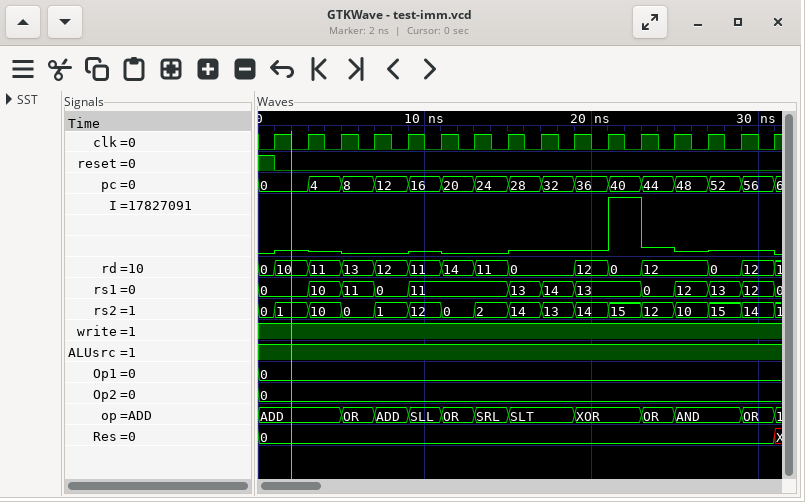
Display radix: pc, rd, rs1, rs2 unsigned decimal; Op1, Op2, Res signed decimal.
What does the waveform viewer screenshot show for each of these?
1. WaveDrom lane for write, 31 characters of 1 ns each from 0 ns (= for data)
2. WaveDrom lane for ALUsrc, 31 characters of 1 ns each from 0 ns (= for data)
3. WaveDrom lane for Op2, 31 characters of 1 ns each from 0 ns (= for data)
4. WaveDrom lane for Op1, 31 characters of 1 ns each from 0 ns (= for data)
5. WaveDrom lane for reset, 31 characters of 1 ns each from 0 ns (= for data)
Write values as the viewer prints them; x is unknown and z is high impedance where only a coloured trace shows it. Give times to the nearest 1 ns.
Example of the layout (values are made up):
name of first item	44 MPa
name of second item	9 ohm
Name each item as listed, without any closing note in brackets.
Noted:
WaveDrom lane for write, 31 characters of 1 ns each from 0 ns	{name: 'write', wave: '1..............................'}
WaveDrom lane for ALUsrc, 31 characters of 1 ns each from 0 ns	{name: 'ALUsrc', wave: '1..............................'}
WaveDrom lane for Op2, 31 characters of 1 ns each from 0 ns	{name: 'Op2', wave: '=..............................', data: '0'}
WaveDrom lane for Op1, 31 characters of 1 ns each from 0 ns	{name: 'Op1', wave: '=..............................', data: '0'}
WaveDrom lane for reset, 31 characters of 1 ns each from 0 ns	{name: 'reset', wave: '10.............................'}
